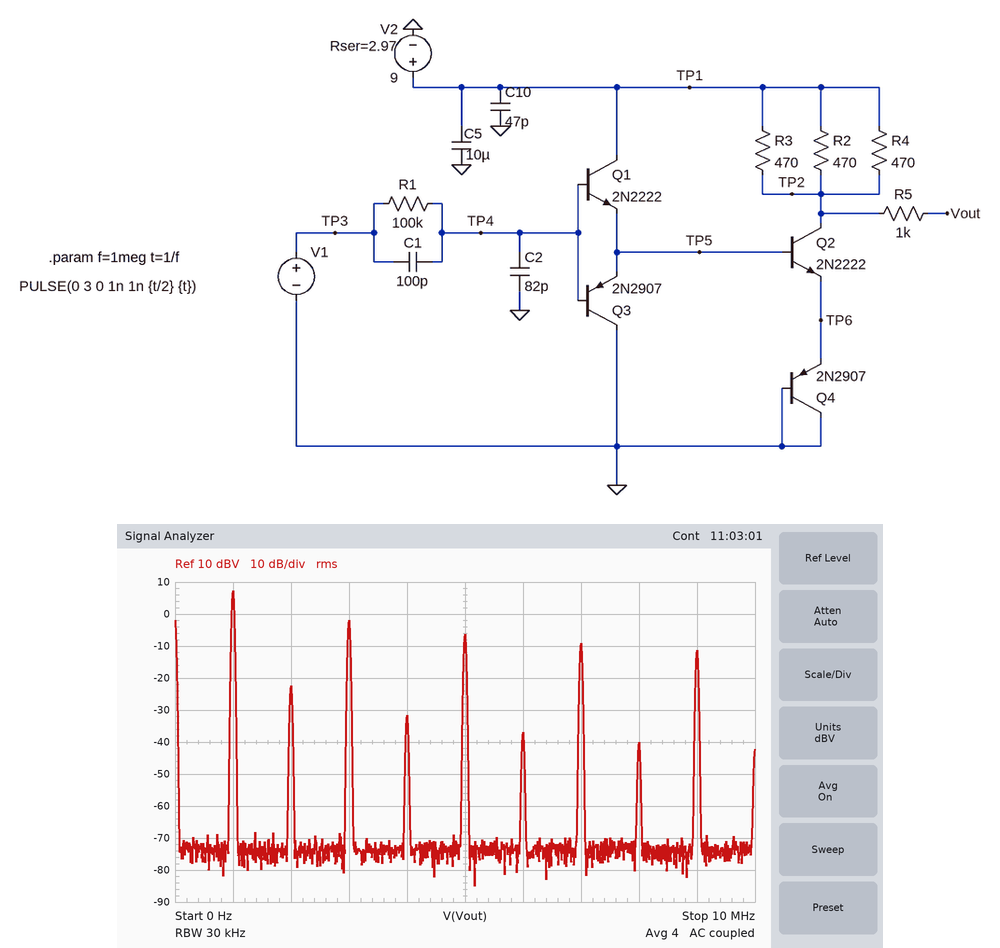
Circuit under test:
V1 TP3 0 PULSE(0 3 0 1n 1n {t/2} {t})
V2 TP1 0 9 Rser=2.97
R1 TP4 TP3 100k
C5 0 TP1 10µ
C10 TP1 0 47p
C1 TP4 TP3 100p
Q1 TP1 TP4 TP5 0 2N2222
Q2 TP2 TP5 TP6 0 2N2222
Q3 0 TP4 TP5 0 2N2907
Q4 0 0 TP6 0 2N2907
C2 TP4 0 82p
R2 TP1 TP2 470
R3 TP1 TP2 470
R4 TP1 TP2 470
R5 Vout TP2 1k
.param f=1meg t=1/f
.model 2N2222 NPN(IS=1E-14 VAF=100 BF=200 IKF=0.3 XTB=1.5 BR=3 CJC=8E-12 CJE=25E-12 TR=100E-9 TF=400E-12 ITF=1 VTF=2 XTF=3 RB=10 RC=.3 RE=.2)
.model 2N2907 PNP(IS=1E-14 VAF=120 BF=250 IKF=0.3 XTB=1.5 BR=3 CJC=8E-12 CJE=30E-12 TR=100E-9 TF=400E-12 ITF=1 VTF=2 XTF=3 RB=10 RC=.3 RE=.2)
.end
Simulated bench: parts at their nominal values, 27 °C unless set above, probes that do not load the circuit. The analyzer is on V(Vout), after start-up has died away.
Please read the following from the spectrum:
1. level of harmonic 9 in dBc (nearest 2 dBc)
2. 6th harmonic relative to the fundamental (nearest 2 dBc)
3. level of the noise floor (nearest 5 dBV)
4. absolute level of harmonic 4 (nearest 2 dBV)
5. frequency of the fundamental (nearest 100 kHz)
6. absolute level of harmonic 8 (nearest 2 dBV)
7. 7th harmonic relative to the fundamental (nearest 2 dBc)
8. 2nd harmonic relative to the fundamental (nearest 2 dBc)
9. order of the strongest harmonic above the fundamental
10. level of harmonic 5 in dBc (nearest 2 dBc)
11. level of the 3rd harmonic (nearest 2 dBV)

-18 dBc
-44 dBc
-75 dBV
-32 dBV
1.0 MHz
-40 dBV
-16 dBc
-30 dBc
3
-14 dBc
-2 dBV
